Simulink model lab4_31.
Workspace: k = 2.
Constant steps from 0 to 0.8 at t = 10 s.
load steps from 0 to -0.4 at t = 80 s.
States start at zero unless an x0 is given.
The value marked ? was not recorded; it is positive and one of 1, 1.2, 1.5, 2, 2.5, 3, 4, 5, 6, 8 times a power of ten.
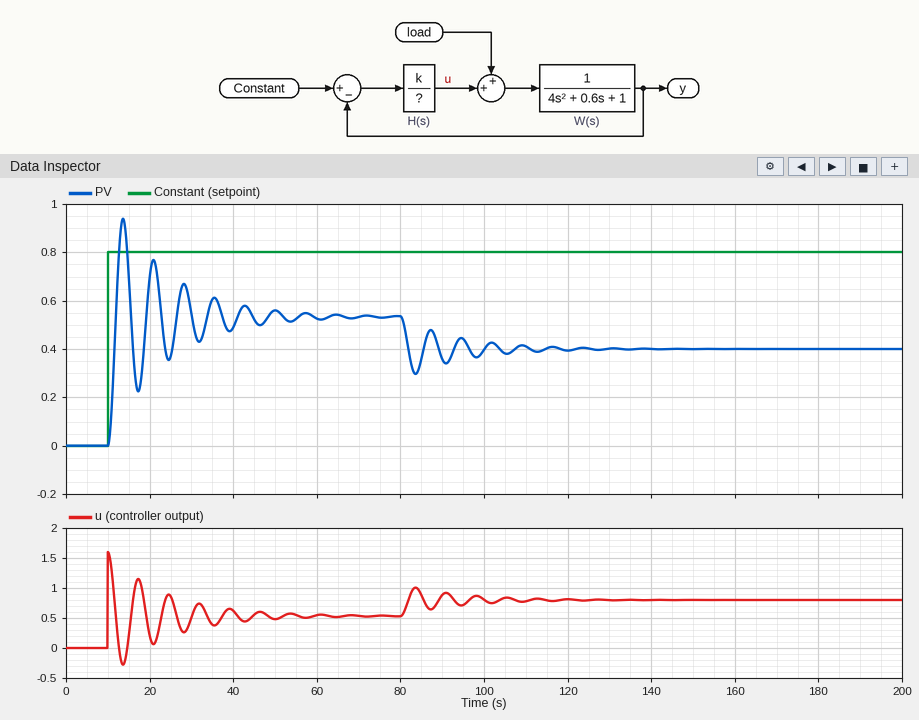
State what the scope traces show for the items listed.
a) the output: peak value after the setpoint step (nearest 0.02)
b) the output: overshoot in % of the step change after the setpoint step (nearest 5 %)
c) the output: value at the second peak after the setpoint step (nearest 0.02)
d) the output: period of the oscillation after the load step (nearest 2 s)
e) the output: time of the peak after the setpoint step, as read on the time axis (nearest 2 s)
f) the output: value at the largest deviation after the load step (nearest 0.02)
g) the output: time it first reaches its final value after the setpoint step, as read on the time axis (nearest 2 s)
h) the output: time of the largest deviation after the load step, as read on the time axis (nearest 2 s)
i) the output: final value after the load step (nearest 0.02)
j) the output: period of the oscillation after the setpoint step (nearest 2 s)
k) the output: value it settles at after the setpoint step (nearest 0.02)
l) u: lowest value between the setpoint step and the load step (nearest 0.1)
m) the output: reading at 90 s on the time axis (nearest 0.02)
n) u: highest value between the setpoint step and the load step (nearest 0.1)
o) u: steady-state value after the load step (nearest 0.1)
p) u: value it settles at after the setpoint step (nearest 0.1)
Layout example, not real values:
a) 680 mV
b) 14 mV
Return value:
a) 0.94
b) 75 %
c) 0.76
d) 8 s
e) 14 s
f) 0.30
g) 12 s
h) 84 s
i) 0.40
j) 8 s
k) 0.54
l) -0.3
m) 0.36
n) 1.6
o) 0.8
p) 0.5
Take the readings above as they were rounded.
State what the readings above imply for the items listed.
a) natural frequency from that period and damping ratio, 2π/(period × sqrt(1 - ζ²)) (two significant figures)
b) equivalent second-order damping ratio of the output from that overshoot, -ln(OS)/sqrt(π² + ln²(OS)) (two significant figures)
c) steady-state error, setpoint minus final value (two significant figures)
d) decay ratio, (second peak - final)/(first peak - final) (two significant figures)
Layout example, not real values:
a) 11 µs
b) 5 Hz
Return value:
a) 0.79 rad/s
b) 0.091
c) 0.26
d) 0.55
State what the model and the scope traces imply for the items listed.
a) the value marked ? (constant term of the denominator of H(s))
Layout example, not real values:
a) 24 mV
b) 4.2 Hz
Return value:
a) 1
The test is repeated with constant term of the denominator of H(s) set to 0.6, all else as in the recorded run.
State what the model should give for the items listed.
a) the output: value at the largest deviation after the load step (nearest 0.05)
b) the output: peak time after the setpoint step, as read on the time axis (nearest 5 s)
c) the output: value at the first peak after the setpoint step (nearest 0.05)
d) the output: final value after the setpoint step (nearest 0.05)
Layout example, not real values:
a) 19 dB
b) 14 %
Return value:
a) 0.45
b) 15 s
c) 1.10
d) 0.60
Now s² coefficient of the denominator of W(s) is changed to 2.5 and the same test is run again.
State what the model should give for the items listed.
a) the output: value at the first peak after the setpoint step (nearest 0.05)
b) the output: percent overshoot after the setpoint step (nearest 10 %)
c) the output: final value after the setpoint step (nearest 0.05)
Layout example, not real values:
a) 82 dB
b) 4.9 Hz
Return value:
a) 0.90
b) 70 %
c) 0.55
